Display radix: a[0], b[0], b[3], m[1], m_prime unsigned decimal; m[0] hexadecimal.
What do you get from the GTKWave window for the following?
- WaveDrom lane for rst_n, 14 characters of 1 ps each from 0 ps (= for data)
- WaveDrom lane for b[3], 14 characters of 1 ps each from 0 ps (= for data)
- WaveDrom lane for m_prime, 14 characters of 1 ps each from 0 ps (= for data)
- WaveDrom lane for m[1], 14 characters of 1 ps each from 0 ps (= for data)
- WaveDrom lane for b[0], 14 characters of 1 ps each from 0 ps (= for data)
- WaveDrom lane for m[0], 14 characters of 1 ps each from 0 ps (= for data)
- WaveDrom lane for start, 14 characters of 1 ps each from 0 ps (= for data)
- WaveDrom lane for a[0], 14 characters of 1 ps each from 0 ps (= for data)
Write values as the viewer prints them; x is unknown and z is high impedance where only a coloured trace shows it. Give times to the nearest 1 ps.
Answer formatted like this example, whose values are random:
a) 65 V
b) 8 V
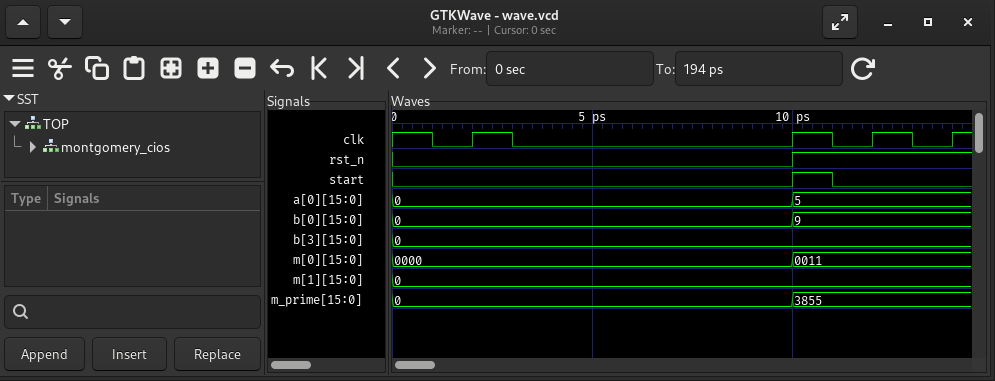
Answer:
a) {name: 'rst_n', wave: '0.........1...'}
b) {name: 'b[3]', wave: '=.............', data: '0'}
c) {name: 'm_prime', wave: '=.........=...', data: '0 3855'}
d) {name: 'm[1]', wave: '=.............', data: '0'}
e) {name: 'b[0]', wave: '=.........=...', data: '0 9'}
f) {name: 'm[0]', wave: '=.........=...', data: '0000 0011'}
g) {name: 'start', wave: '0.........10..'}
h) {name: 'a[0]', wave: '=.........=...', data: '0 5'}
